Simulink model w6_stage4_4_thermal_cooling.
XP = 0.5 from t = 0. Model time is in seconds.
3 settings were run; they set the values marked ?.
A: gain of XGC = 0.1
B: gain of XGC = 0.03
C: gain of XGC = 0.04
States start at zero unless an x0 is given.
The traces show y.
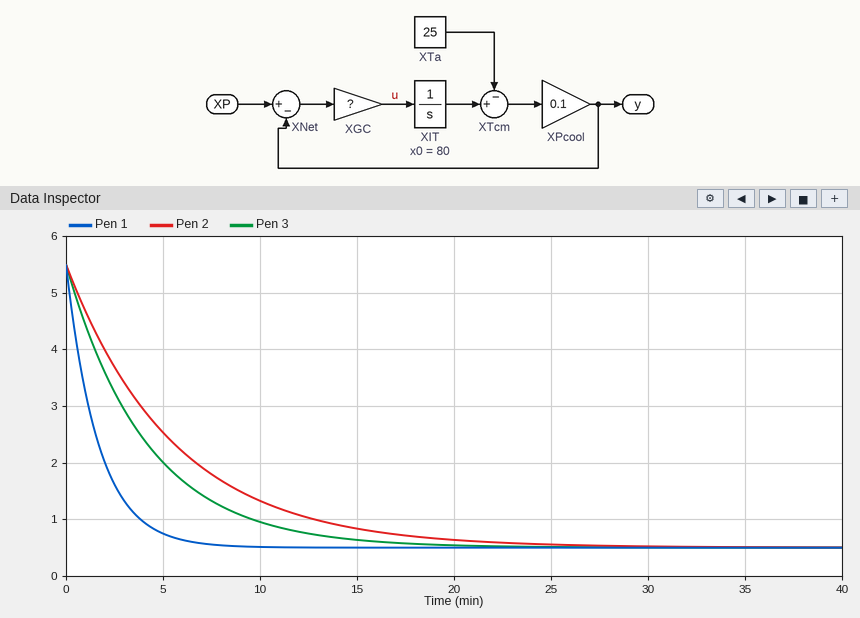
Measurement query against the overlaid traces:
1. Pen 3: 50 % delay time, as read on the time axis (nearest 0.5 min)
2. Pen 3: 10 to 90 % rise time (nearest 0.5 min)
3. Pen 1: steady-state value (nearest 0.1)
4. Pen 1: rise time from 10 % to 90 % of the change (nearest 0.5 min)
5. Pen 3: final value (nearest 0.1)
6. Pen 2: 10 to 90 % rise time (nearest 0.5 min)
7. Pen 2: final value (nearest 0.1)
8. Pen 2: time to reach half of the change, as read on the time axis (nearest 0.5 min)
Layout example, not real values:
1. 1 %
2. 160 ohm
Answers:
1. 3.0 min
2. 9.0 min
3. 0.5
4. 3.5 min
5. 0.5
6. 12.0 min
7. 0.5
8. 4.0 min
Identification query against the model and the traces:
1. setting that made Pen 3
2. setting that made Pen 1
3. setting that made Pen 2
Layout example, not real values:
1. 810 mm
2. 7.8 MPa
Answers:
1. C
2. A
3. B
